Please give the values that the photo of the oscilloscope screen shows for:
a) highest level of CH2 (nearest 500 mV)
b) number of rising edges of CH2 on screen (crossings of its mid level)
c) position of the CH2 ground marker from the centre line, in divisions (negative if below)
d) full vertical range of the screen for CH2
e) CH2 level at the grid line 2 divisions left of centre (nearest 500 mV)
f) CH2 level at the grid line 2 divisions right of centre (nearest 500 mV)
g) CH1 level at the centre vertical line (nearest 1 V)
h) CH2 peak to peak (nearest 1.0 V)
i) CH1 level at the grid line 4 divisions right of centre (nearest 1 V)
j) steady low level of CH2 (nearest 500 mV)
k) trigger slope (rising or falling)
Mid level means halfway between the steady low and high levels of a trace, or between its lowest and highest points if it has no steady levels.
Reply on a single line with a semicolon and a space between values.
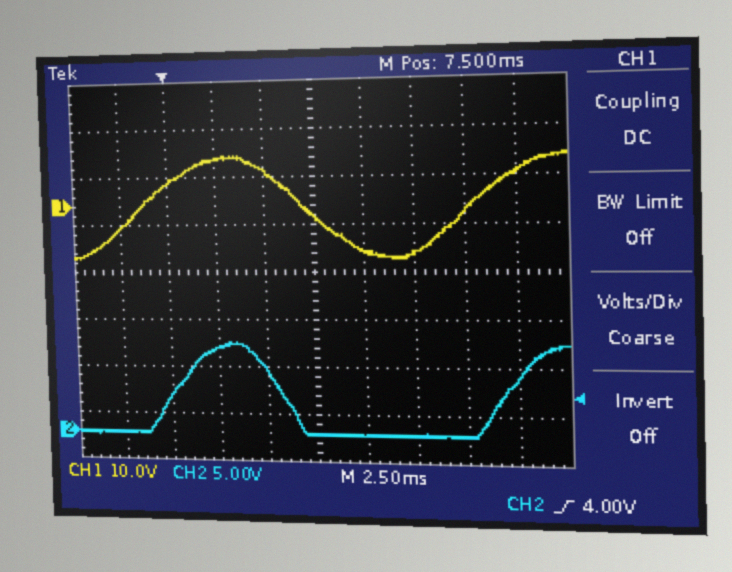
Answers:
9.5 V; 2; -3.4 div; 40 V; 9.0 V; 0.0 V; -2 V; 10.0 V; 7 V; 0.0 V; rising
